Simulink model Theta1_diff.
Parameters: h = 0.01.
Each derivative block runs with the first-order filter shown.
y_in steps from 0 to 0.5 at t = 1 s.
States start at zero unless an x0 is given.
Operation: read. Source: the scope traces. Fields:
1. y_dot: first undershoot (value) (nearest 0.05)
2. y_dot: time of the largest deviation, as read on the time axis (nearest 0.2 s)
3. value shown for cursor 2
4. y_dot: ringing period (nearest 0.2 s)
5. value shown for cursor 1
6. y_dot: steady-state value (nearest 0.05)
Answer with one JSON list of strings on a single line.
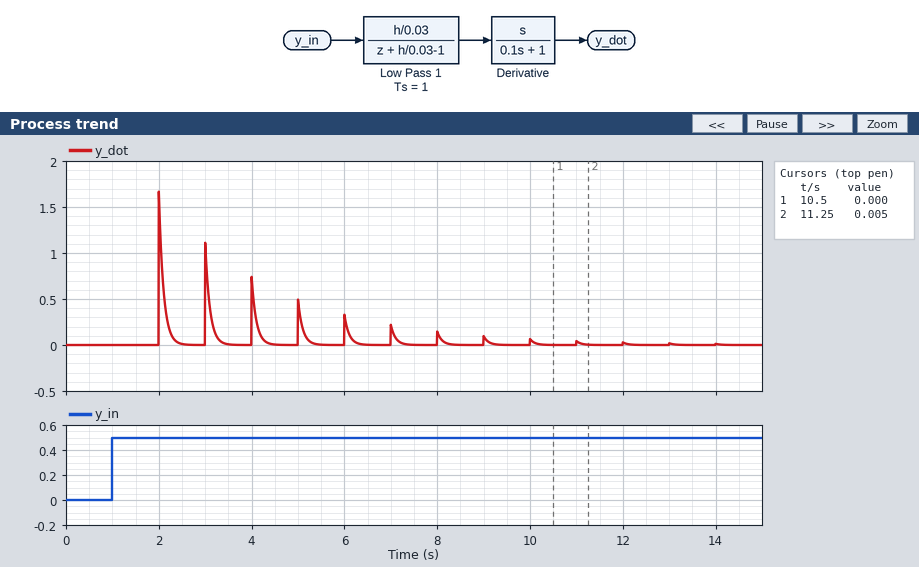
["0.00", "2.0 s", "0.005", "1.0 s", "0.000", "0.00"]
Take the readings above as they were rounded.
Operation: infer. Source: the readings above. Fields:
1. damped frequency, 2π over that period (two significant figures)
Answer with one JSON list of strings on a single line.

["6.3 rad/s"]
